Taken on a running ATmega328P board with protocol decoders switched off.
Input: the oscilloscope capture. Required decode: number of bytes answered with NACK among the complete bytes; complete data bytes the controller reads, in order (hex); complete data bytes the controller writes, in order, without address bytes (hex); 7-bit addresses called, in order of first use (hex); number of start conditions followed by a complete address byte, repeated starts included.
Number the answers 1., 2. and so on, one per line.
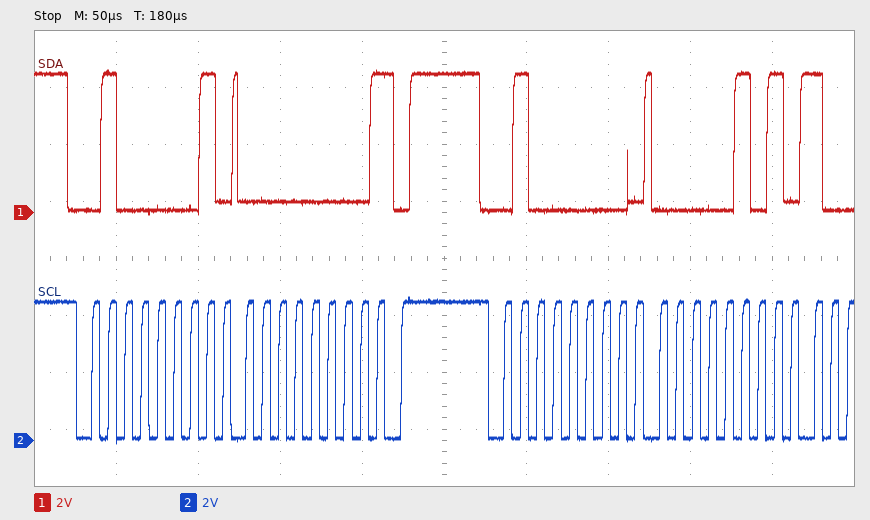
1. 1
2. 00
3. 05
4. 0x20
5. 2
